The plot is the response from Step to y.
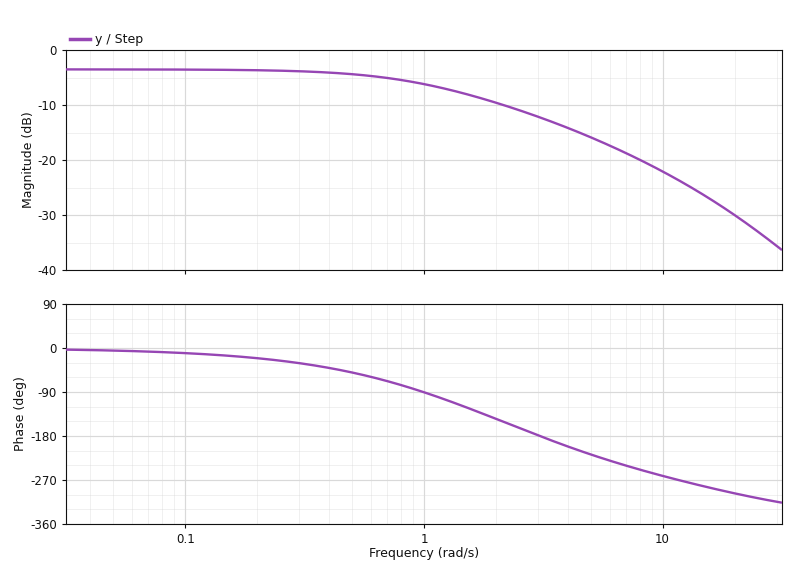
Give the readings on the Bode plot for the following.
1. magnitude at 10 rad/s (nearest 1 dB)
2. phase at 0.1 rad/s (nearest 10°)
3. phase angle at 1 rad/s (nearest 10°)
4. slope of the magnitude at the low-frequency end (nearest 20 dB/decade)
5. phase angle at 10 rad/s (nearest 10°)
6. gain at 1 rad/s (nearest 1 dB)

-22 dB
-10°
-90°
0 dB/decade
-260°
-6 dB
